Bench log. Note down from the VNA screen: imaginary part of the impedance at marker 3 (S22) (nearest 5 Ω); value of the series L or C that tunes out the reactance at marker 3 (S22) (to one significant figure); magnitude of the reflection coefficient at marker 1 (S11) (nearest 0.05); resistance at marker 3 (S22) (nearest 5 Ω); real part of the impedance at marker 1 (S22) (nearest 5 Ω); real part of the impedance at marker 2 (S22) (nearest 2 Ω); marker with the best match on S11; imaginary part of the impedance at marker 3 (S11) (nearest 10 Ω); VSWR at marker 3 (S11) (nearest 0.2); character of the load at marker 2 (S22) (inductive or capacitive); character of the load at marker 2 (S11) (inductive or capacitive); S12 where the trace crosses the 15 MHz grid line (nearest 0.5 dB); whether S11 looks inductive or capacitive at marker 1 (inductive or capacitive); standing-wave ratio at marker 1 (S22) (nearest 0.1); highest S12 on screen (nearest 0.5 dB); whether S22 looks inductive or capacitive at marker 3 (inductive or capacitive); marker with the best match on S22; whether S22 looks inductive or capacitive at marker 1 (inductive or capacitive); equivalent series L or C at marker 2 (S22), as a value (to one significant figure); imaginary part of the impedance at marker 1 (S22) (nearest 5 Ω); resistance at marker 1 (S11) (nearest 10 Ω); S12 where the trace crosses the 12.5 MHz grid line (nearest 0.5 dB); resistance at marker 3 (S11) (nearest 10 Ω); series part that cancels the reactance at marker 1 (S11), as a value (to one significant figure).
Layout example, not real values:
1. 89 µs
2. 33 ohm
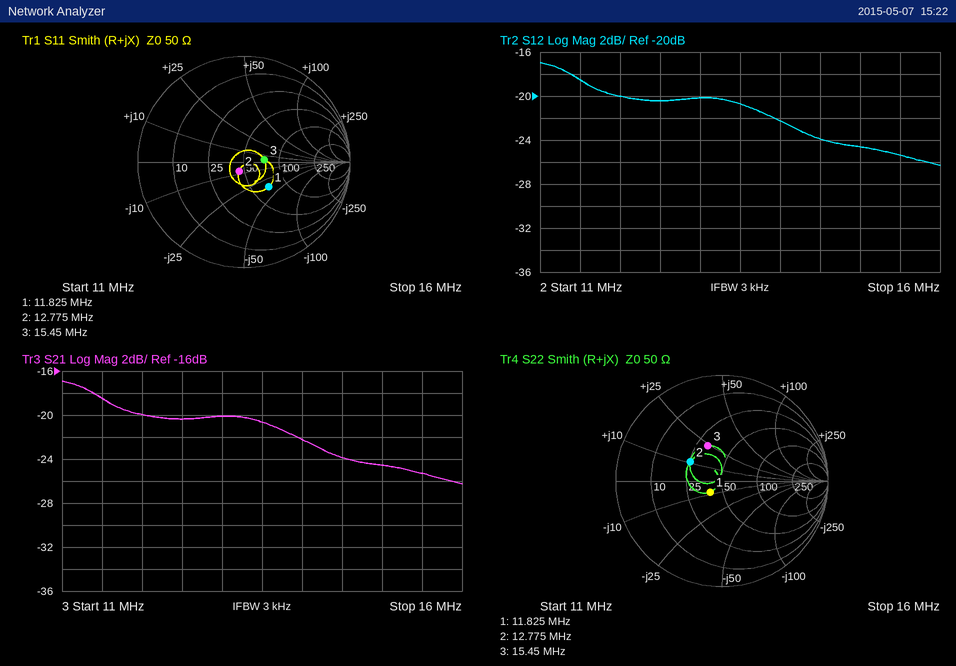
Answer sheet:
1. +25 Ω
2. 400 pF
3. 0.35
4. 30 Ω
5. 40 Ω
6. 26 Ω
7. marker 2
8. 0 Ω
9. 1.4
10. inductive
11. capacitive
12. -24.5 dB
13. capacitive
14. 1.4
15. -17.0 dB
16. inductive
17. marker 1
18. capacitive
19. 100 nH
20. -10 Ω
21. 70 Ω
22. -20.5 dB
23. 70 Ω
24. 500 nH
